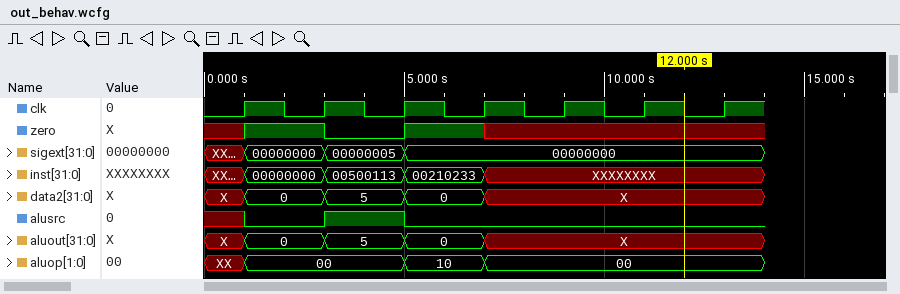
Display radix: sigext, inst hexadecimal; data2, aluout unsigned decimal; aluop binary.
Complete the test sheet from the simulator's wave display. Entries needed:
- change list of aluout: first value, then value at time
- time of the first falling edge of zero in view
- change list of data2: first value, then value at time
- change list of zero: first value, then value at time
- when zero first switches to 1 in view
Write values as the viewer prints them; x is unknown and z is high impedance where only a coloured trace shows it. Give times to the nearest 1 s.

X, 0 at 1 s, 5 at 3 s, 0 at 5 s, X at 7 s
3 s
X, 0 at 1 s, 5 at 3 s, 0 at 5 s, X at 7 s
x, 1 at 1 s, 0 at 3 s, 1 at 5 s, x at 7 s
1 s
